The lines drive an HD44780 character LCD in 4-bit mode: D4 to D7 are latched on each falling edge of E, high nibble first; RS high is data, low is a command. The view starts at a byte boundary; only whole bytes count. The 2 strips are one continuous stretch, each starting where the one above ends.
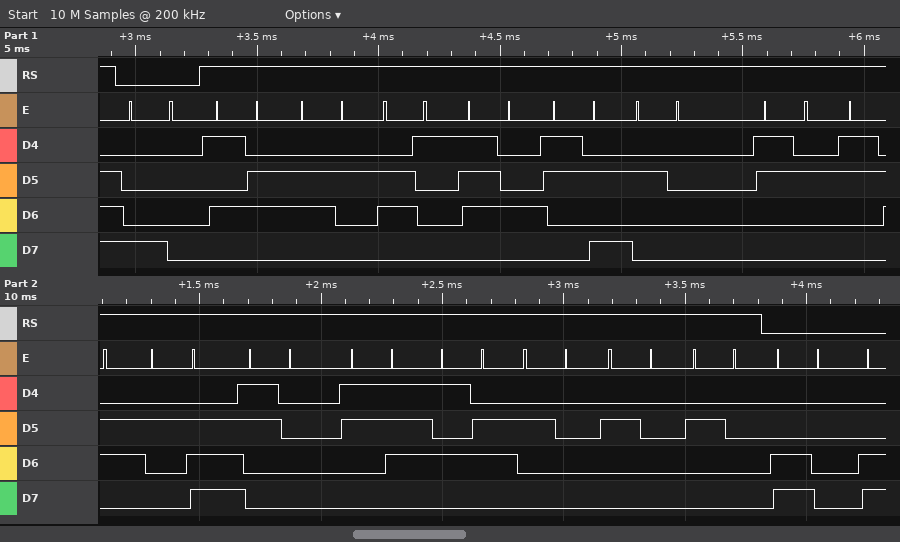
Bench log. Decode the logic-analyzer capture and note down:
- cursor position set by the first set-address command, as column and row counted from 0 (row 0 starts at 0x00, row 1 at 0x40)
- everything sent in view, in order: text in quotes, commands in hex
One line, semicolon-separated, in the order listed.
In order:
column 0, row 0; 0x80 "Vbat: 26.07V   " 0xC0
